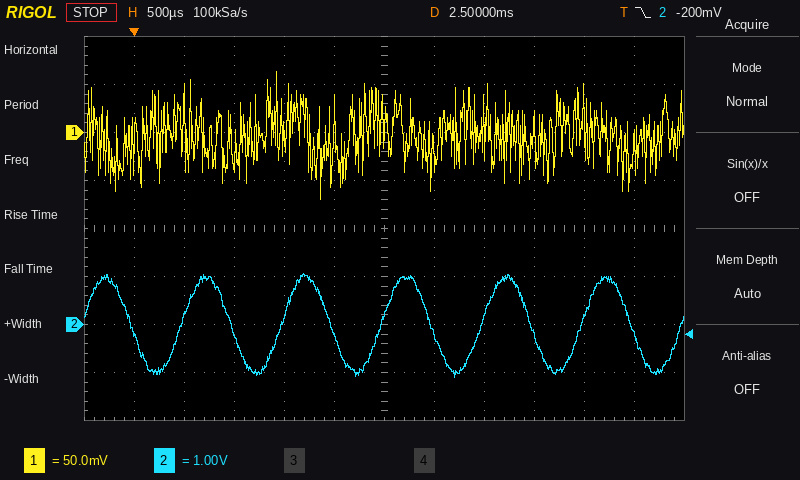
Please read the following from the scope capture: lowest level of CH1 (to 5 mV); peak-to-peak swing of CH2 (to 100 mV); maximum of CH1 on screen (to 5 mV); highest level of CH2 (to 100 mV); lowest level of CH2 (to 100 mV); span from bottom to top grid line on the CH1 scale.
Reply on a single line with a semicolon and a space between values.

-70 mV; 2.2 V; 65 mV; 1.1 V; -1.1 V; 400 mV
